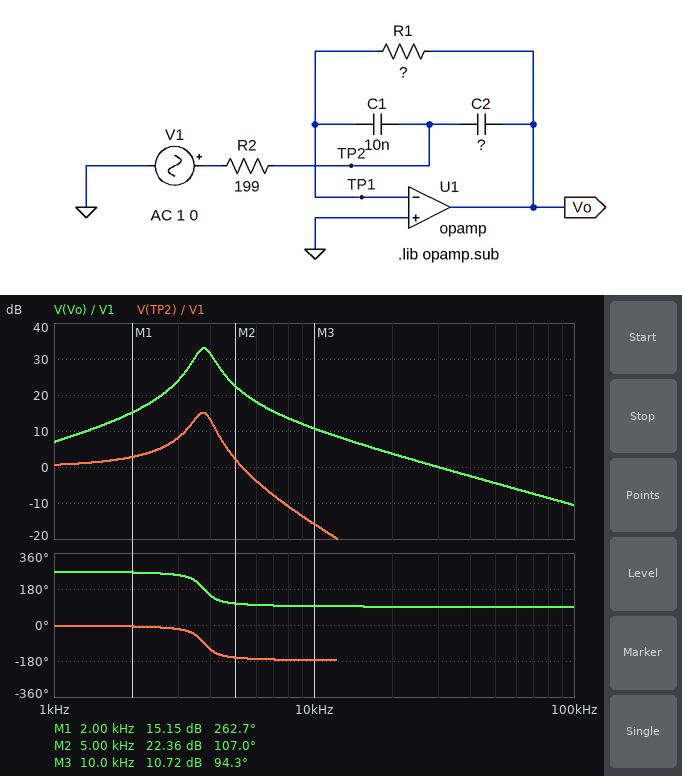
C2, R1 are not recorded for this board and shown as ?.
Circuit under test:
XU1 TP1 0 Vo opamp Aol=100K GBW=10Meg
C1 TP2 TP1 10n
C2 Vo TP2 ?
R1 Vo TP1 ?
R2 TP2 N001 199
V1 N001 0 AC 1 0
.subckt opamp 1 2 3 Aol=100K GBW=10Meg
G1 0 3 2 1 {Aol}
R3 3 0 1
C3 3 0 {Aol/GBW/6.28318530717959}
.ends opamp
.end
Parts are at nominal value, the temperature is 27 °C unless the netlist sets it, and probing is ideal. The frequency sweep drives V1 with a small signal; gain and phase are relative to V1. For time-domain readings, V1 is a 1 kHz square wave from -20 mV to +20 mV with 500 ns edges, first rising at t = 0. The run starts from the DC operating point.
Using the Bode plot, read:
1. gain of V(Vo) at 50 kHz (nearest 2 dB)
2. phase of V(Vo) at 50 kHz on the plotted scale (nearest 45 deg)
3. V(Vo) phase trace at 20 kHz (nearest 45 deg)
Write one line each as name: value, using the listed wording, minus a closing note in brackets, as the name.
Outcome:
gain of V(Vo) at 50 kHz: -4 dB
phase of V(Vo) at 50 kHz on the plotted scale: 90 deg
V(Vo) phase trace at 20 kHz: 90 deg
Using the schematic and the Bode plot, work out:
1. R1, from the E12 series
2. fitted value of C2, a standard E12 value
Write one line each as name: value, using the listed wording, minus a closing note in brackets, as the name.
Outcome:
R1, from the E12 series: 33 kΩ
fitted value of C2, a standard E12 value: 27 nF
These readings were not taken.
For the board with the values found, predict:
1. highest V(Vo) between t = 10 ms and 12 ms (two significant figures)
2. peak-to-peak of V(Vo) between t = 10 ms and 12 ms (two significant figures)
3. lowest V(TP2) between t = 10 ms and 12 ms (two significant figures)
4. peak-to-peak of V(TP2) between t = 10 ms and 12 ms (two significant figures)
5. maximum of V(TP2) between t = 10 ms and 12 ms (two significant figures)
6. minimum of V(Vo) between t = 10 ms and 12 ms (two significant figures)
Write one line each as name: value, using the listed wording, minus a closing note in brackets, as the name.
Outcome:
highest V(Vo) between t = 10 ms and 12 ms: 220 mV
peak-to-peak of V(Vo) between t = 10 ms and 12 ms: 440 mV
lowest V(TP2) between t = 10 ms and 12 ms: -44 mV
peak-to-peak of V(TP2) between t = 10 ms and 12 ms: 88 mV
maximum of V(TP2) between t = 10 ms and 12 ms: 44 mV
minimum of V(Vo) between t = 10 ms and 12 ms: -220 mV
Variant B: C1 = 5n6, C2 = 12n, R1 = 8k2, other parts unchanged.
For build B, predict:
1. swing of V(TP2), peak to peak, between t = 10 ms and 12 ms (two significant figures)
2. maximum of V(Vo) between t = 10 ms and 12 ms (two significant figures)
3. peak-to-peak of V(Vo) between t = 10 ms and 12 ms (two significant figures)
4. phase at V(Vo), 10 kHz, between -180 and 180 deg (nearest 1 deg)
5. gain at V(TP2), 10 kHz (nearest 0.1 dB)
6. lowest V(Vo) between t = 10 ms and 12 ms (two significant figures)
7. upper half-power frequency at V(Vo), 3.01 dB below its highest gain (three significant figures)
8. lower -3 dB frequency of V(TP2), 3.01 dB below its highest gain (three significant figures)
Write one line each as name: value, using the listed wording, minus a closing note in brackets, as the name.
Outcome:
swing of V(TP2), peak to peak, between t = 10 ms and 12 ms: 87 mV
maximum of V(Vo) between t = 10 ms and 12 ms: 140 mV
peak-to-peak of V(Vo) between t = 10 ms and 12 ms: 280 mV
phase at V(Vo), 10 kHz, between -180 and 180 deg: -111 deg
gain at V(TP2), 10 kHz: 4.3 dB
lowest V(Vo) between t = 10 ms and 12 ms: -140 mV
upper half-power frequency at V(Vo), 3.01 dB below its highest gain: 17.9 kHz
lower -3 dB frequency of V(TP2), 3.01 dB below its highest gain: 11.9 kHz
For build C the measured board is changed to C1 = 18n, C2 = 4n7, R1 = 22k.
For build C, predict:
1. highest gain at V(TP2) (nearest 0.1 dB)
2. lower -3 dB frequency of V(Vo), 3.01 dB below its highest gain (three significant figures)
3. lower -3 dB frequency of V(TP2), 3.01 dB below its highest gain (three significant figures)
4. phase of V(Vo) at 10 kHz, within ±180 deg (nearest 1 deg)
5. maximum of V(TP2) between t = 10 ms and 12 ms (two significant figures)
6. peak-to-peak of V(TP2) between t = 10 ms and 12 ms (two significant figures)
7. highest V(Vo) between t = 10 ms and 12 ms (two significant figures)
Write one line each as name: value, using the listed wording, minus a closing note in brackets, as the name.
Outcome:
highest gain at V(TP2): 12.6 dB
lower -3 dB frequency of V(Vo), 3.01 dB below its highest gain: 7.30 kHz
lower -3 dB frequency of V(TP2), 3.01 dB below its highest gain: 7.05 kHz
phase of V(Vo) at 10 kHz, within ±180 deg: 120 deg
maximum of V(TP2) between t = 10 ms and 12 ms: 46 mV
peak-to-peak of V(TP2) between t = 10 ms and 12 ms: 92 mV
highest V(Vo) between t = 10 ms and 12 ms: 660 mV
